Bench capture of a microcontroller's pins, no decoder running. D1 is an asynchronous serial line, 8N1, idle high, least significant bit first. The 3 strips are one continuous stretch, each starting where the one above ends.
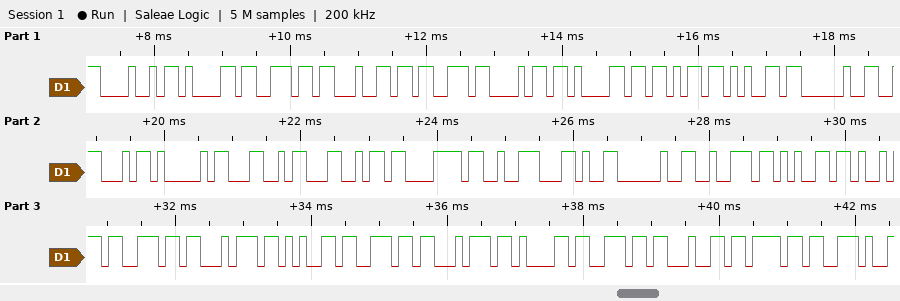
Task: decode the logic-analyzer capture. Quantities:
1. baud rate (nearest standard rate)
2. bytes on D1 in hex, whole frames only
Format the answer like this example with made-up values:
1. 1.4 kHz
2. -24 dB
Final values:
1. 9600 baud
2. 48 61 6E 64 73 68 61 6B 65 20 46 41 4C 4C C3 93 2C 20 72 65 69 6E 74 65 6E 74 61 6E 64 6F 2E
